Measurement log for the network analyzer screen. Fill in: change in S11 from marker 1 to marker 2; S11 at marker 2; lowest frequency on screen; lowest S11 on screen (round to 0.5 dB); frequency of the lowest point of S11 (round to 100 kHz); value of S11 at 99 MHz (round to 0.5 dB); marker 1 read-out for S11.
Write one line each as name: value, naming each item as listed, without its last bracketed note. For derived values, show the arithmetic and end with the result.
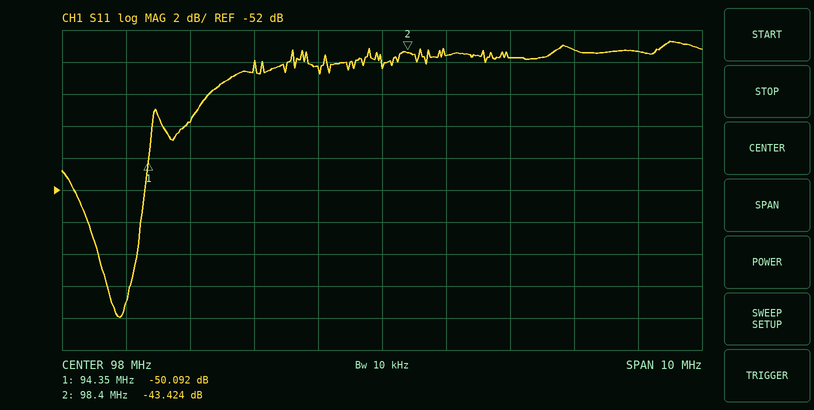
change in S11 from marker 1 to marker 2: -43.424 − (-50.092) = 6.668 dB
S11 at marker 2: -43.424 dB
lowest frequency on screen: 93 MHz
lowest S11 on screen: -60.0 dB
frequency of the lowest point of S11: 93.9 MHz
value of S11 at 99 MHz: -43.5 dB
marker 1 read-out for S11: -50.092 dB
